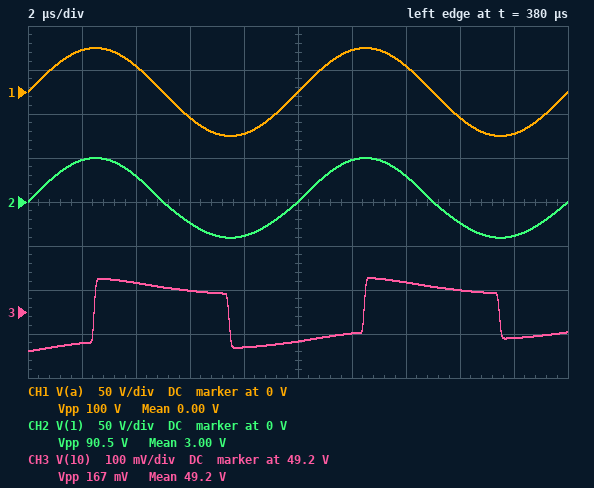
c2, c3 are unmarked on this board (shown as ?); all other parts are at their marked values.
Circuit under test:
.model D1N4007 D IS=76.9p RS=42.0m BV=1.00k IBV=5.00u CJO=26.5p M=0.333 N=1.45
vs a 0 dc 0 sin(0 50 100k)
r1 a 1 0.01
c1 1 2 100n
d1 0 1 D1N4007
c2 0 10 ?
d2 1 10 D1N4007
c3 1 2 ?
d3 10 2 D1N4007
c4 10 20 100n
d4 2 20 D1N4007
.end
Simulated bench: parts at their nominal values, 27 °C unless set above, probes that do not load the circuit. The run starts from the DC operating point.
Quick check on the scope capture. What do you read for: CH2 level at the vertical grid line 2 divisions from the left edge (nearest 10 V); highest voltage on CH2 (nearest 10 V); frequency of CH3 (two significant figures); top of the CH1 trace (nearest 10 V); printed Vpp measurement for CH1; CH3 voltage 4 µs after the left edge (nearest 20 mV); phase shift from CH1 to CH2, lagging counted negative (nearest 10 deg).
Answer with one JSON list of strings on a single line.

["30 V", "50 V", "100 kHz", "50 V", "100 V", "49.26 V", "0 deg"]
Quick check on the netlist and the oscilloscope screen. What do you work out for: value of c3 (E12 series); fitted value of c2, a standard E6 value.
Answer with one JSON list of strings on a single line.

["150 nF", "68 nF"]
